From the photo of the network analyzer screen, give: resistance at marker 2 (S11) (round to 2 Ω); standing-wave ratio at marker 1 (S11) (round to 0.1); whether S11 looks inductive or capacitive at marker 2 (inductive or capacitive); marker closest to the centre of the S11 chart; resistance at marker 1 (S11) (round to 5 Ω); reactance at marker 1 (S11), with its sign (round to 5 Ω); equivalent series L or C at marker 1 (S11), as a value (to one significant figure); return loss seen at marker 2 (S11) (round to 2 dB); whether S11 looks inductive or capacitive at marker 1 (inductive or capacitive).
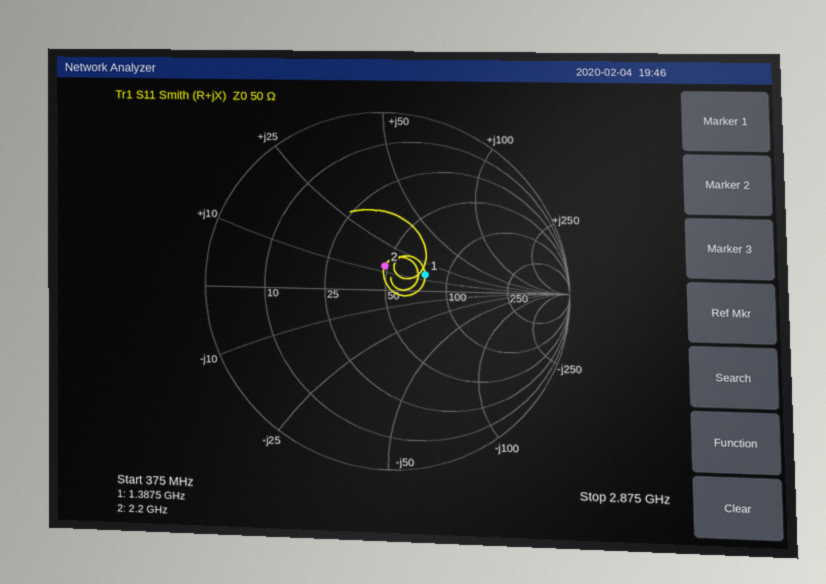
48 Ω
1.6
inductive
marker 2
75 Ω
+15 Ω
2 nH
18 dB
inductive
